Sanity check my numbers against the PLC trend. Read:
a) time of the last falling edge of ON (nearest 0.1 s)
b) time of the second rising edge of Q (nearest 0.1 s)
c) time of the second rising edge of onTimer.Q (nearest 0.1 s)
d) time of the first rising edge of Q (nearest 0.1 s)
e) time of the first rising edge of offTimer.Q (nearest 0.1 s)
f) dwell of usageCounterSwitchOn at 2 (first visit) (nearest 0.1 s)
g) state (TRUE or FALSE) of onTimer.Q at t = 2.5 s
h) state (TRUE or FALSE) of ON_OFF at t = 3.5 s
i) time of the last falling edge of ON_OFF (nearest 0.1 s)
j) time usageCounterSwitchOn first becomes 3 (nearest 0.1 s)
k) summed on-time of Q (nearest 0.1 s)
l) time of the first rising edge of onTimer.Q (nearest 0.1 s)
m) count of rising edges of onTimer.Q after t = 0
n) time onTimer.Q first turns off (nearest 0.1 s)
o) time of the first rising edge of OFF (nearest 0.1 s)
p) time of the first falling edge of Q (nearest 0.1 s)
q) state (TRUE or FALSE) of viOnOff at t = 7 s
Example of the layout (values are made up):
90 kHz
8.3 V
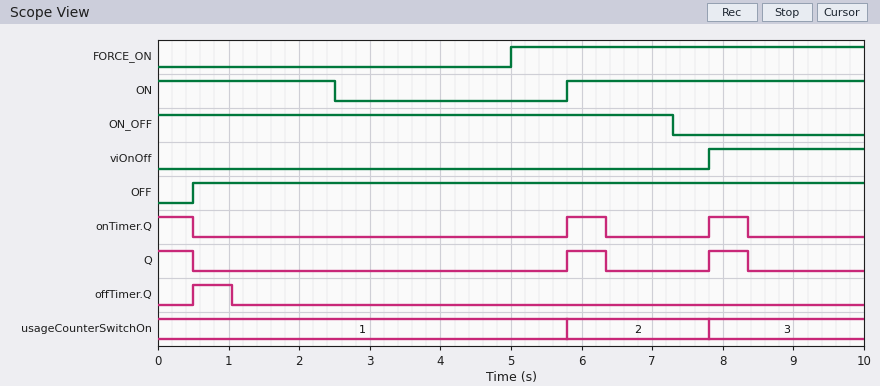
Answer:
2.5 s
7.8 s
7.8 s
5.8 s
0.5 s
2.0 s
FALSE
TRUE
7.3 s
7.8 s
1.6 s
5.8 s
2
0.5 s
0.5 s
0.5 s
FALSE
